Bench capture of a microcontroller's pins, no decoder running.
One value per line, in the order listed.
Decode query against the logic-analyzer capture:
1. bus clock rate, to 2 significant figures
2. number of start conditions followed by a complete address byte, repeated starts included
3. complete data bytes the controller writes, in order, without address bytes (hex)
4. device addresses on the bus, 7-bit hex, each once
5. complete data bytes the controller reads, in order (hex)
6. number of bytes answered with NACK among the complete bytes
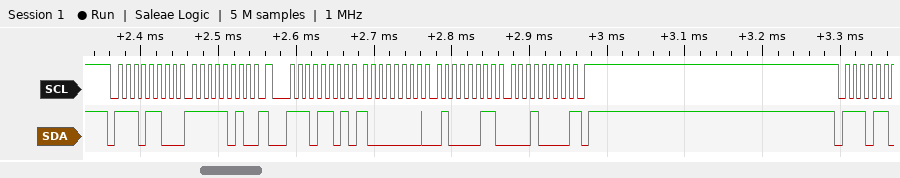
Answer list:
100 kHz
2
FA
0x76
80 43 10
1
